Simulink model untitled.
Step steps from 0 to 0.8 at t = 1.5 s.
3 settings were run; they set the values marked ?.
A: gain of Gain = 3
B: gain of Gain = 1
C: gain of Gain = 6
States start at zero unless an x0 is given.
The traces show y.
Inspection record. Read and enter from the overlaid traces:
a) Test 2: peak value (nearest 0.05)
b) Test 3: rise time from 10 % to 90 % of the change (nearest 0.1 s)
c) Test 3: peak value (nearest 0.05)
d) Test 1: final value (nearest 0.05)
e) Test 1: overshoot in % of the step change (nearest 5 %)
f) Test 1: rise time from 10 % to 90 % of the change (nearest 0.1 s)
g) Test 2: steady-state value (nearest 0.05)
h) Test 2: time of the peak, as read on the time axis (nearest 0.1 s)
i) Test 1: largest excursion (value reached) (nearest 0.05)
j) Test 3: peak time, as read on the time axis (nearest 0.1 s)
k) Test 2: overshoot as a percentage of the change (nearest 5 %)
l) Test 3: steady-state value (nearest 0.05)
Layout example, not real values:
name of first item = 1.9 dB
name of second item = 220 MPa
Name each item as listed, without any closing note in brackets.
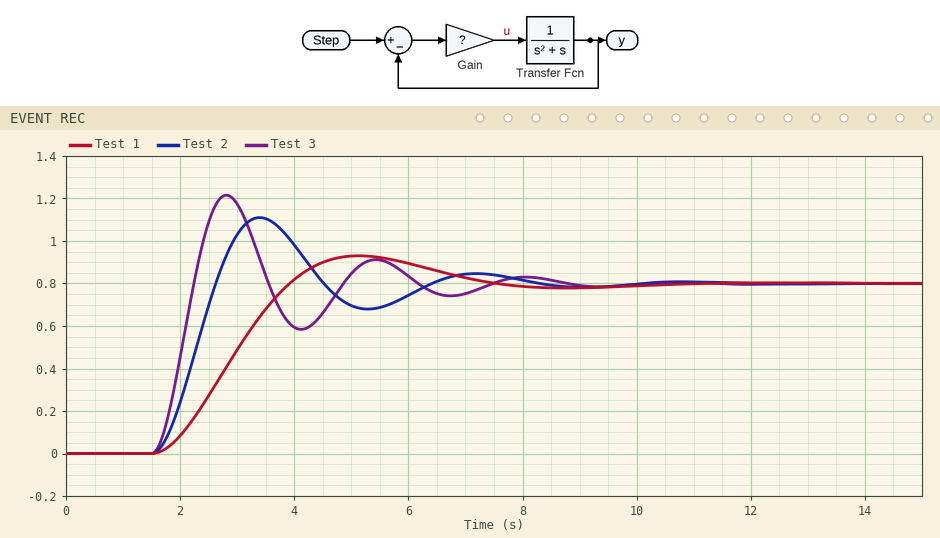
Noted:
Test 2: peak value = 1.10
Test 3: rise time from 10 % to 90 % of the change = 0.5 s
Test 3: peak value = 1.20
Test 1: final value = 0.80
Test 1: overshoot in % of the step change = 15 %
Test 1: rise time from 10 % to 90 % of the change = 1.6 s
Test 2: steady-state value = 0.80
Test 2: time of the peak, as read on the time axis = 3.4 s
Test 1: largest excursion (value reached) = 0.95
Test 3: peak time, as read on the time axis = 2.8 s
Test 2: overshoot as a percentage of the change = 40 %
Test 3: steady-state value = 0.80
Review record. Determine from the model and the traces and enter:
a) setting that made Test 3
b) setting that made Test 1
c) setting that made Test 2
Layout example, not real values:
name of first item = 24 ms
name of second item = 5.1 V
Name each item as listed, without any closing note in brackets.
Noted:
setting that made Test 3 = C
setting that made Test 1 = B
setting that made Test 2 = A
